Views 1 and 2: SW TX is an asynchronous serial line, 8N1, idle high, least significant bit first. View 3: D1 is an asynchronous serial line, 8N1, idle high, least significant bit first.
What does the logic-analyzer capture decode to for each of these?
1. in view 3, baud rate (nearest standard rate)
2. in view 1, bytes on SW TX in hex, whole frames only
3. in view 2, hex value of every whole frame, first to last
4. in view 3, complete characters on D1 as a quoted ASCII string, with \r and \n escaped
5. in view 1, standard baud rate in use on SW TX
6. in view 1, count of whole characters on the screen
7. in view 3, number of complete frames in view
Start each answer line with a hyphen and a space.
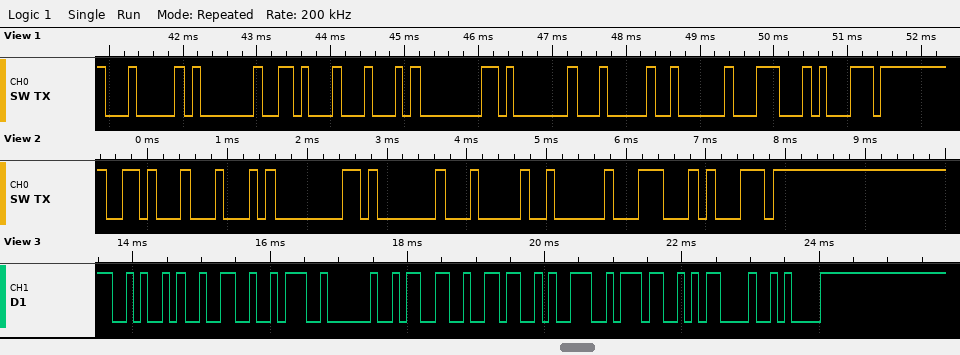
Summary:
- 9600 baud
- 04 01 16 44 80 01 04 02 1C 71
- 16 44 80 01 04 02 1C 71
- "J2: 3697\r\n"
- 9600 baud
- 10
- 10
